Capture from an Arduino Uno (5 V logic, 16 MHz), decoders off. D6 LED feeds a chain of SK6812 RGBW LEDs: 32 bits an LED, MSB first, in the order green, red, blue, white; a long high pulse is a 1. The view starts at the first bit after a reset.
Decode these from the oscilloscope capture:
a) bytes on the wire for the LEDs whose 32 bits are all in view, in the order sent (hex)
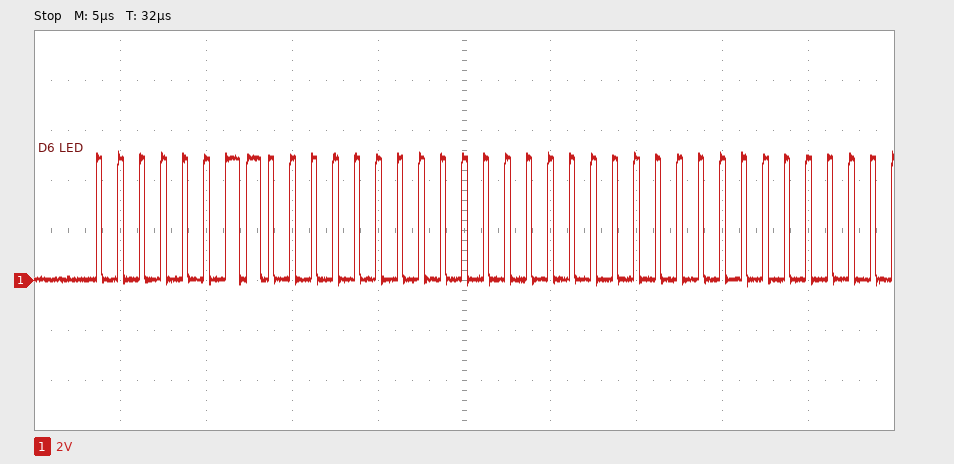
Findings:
03 00 00 00
